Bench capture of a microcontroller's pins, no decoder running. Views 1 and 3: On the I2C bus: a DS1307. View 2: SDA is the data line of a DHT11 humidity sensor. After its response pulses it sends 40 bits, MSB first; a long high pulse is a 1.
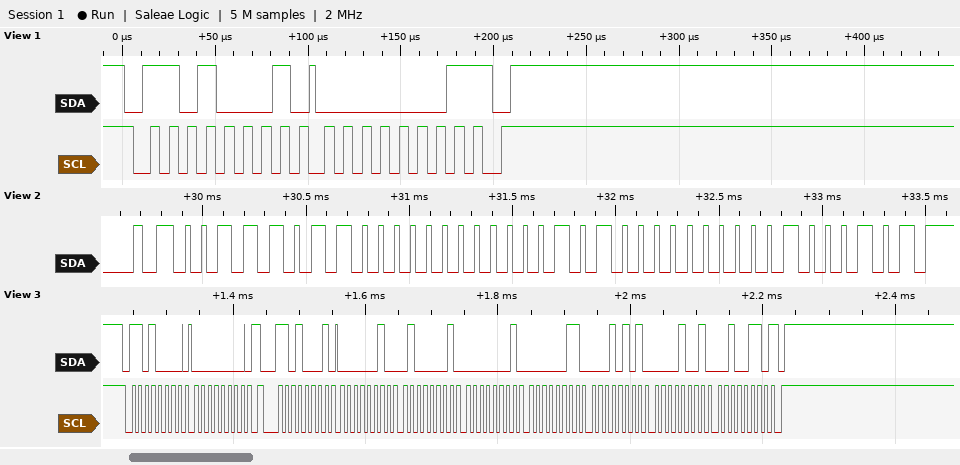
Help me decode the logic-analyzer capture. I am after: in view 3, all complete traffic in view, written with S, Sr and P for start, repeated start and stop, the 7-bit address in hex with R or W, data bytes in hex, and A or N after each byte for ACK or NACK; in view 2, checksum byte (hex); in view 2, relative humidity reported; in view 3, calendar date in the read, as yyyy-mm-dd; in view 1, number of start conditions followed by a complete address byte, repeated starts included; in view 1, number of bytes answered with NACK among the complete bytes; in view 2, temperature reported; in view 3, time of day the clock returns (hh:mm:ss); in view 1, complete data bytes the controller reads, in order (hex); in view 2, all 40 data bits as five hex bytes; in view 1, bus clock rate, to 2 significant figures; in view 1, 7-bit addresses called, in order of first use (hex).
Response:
S 68W A 00 A Sr 68R A 02 A 41 A 01 A 03 A 15 A 09 A 26 N P
0x45
59 %
2026-09-15
1
1
10.0 °C
01:41:02
01
3B 00 0A 00 45
100 kHz
0x68
